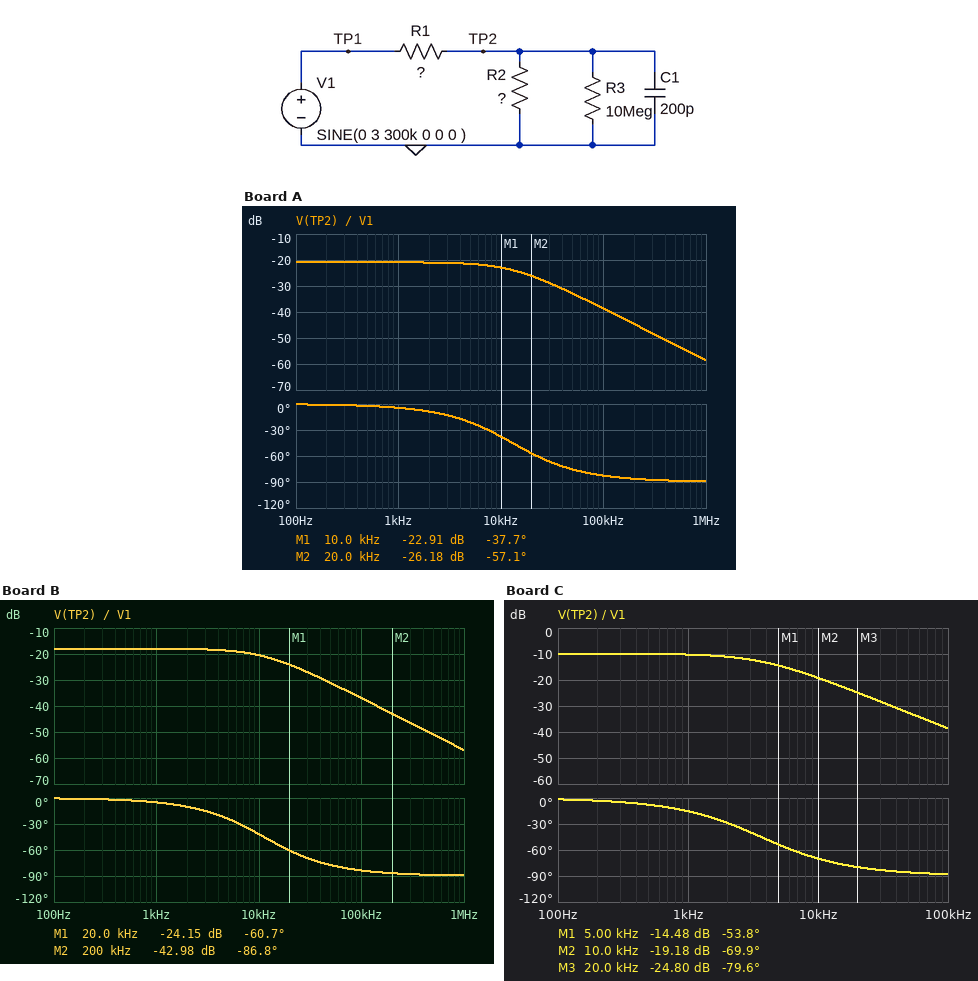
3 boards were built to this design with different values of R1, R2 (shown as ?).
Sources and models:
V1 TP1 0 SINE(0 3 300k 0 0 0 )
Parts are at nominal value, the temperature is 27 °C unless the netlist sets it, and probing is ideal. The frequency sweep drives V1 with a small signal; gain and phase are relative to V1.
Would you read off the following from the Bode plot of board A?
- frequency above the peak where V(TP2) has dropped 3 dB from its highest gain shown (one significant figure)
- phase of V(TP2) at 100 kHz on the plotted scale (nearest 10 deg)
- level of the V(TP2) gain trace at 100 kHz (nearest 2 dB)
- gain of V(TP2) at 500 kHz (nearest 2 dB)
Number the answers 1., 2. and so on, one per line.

1. 10 kHz
2. -80 deg
3. -38 dB
4. -52 dB
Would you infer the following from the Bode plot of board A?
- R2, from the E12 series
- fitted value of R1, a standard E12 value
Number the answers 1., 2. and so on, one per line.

1. 68 kΩ
2. 680 kΩ
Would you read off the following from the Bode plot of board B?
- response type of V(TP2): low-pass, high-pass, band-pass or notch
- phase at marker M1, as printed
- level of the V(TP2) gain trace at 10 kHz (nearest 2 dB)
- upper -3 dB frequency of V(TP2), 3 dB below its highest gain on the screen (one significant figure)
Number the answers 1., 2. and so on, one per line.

1. low-pass
2. -60.7 deg
3. -20 dB
4. 10 kHz
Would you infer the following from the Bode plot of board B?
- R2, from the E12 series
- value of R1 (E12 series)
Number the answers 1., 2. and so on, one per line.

1. 82 kΩ
2. 560 kΩ
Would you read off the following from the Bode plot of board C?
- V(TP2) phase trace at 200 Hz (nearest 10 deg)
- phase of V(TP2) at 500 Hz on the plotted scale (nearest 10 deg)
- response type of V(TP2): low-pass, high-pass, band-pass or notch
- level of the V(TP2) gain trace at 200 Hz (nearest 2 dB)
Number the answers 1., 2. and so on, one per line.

1. 0 deg
2. -10 deg
3. low-pass
4. -10 dB
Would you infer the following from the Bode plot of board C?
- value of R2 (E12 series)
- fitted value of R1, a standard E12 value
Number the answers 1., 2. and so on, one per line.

1. 330 kΩ
2. 680 kΩ
